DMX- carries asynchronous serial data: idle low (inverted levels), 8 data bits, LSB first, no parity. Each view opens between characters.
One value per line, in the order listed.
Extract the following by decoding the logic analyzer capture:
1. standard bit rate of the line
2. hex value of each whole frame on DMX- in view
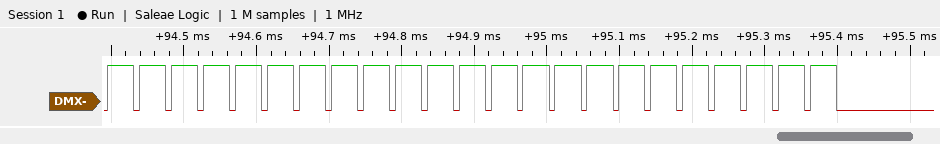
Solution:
115200 baud
08, 08, 08, 08, 08, 08, 08, 08, 08, 08, 08, F8
